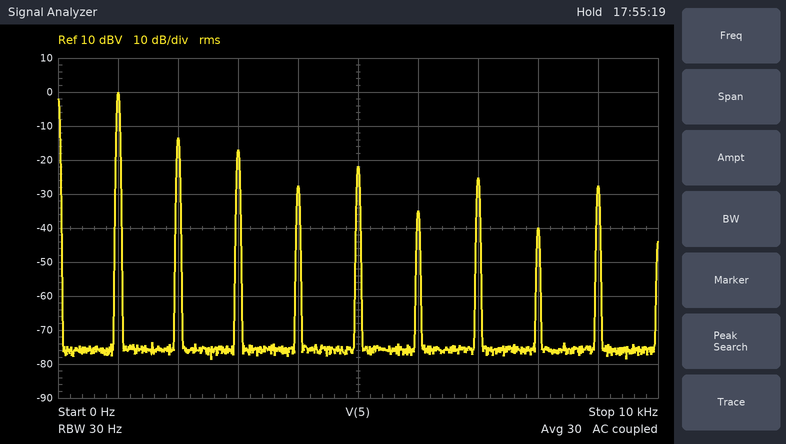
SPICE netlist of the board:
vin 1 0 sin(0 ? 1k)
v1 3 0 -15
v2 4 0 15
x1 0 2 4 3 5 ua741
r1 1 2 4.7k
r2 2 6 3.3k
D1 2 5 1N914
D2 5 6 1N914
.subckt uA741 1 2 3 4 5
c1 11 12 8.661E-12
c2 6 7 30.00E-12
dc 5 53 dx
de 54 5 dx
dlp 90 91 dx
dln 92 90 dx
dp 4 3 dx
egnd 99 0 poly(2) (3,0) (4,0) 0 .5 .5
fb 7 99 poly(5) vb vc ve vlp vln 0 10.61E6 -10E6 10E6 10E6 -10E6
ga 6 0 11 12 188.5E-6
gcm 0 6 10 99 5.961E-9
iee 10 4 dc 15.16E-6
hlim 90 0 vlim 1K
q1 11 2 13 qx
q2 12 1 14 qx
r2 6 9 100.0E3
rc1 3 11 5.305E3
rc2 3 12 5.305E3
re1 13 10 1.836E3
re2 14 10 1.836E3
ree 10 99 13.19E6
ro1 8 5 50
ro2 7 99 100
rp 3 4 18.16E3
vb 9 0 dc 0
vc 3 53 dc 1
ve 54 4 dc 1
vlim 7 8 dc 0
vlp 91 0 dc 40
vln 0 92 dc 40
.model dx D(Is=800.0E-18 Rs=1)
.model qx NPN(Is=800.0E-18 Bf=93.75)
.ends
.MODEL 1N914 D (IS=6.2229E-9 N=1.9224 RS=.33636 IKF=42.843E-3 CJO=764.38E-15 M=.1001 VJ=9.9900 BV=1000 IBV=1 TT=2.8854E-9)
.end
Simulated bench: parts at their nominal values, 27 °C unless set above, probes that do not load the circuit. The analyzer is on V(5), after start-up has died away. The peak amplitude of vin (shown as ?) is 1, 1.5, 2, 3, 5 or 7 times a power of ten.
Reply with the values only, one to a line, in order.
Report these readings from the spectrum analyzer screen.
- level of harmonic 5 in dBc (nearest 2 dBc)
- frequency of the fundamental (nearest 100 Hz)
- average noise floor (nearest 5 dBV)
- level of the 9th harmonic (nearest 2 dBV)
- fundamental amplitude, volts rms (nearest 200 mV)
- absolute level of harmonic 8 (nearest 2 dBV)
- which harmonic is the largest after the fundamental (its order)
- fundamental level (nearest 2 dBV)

-22 dBc
1.0 kHz
-75 dBV
-28 dBV
1.0 V
-40 dBV
2
0 dBV
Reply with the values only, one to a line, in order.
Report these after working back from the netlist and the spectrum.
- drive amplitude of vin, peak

2 V
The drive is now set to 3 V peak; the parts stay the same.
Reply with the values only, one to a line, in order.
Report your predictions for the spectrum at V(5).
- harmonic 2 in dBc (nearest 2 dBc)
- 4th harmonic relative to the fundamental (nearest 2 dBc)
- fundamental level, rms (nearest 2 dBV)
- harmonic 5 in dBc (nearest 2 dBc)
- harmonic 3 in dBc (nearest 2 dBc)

-12 dBc
-26 dBc
2 dBV
-24 dBc
-18 dBc
